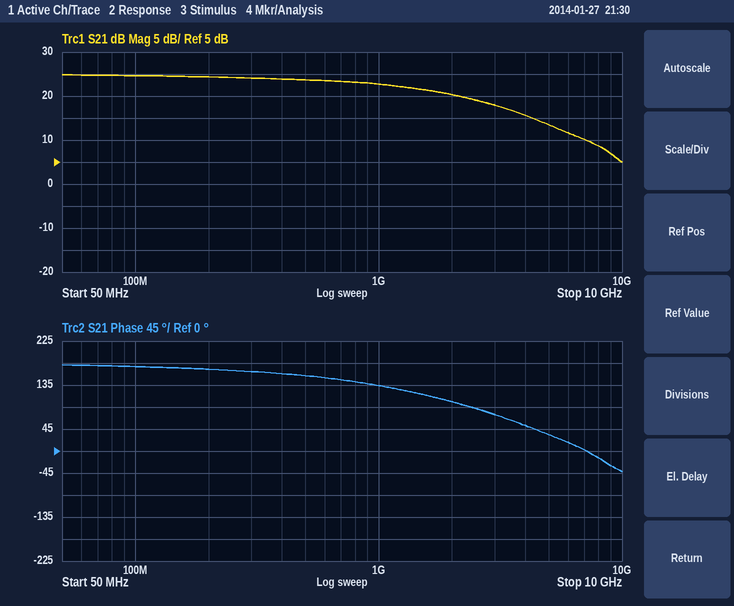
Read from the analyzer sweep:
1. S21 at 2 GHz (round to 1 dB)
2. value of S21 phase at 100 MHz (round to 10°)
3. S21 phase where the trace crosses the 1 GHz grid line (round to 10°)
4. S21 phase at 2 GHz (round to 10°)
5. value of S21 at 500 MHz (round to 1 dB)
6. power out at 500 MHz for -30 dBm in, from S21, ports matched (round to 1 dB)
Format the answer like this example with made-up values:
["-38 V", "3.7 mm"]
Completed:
["20 dB", "170°", "130°", "100°", "24 dB", "-6 dBm"]
